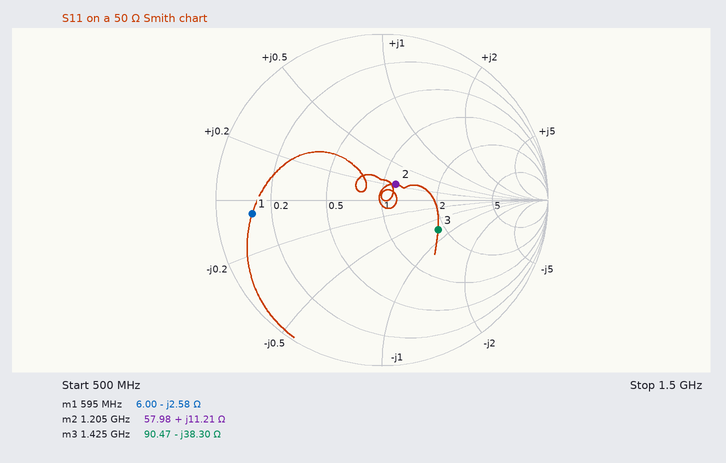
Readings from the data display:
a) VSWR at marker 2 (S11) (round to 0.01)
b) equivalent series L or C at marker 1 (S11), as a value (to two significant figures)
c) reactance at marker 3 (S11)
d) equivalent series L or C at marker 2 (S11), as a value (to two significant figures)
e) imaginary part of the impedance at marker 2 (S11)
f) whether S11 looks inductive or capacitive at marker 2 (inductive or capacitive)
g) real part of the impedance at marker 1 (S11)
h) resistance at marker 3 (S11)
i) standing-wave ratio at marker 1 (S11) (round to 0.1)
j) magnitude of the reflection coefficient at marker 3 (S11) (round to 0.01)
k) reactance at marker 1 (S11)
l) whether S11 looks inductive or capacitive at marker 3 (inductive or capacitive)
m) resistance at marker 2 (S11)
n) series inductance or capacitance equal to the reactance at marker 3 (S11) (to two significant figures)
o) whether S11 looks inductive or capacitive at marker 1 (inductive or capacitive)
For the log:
1.29
100 pF
-38.30 Ω
1.5 nH
+11.21 Ω
inductive
6.00 Ω
90.47 Ω
8.4
0.38
-2.58 Ω
capacitive
57.98 Ω
2.9 pF
capacitive
